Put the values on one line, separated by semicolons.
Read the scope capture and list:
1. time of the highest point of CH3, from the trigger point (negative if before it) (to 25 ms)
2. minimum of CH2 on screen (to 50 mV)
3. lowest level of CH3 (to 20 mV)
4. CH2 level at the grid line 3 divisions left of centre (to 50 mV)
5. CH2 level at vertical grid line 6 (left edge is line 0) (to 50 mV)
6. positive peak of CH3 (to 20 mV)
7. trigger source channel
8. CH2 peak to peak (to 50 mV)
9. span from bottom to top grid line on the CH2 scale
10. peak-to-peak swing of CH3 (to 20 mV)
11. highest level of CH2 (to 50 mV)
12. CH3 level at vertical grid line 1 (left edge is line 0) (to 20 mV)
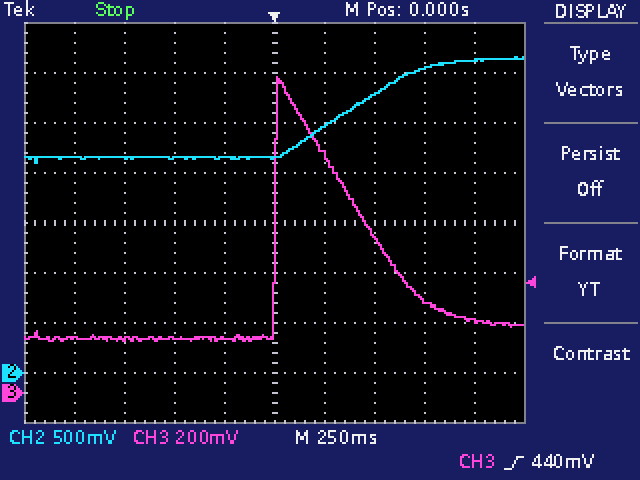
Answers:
+25 ms; 2.10 V; 200 mV; 2.15 V; 2.45 V; 1.26 V; CH3; 1.05 V; 4 V; 1.06 V; 3.15 V; 220 mV
